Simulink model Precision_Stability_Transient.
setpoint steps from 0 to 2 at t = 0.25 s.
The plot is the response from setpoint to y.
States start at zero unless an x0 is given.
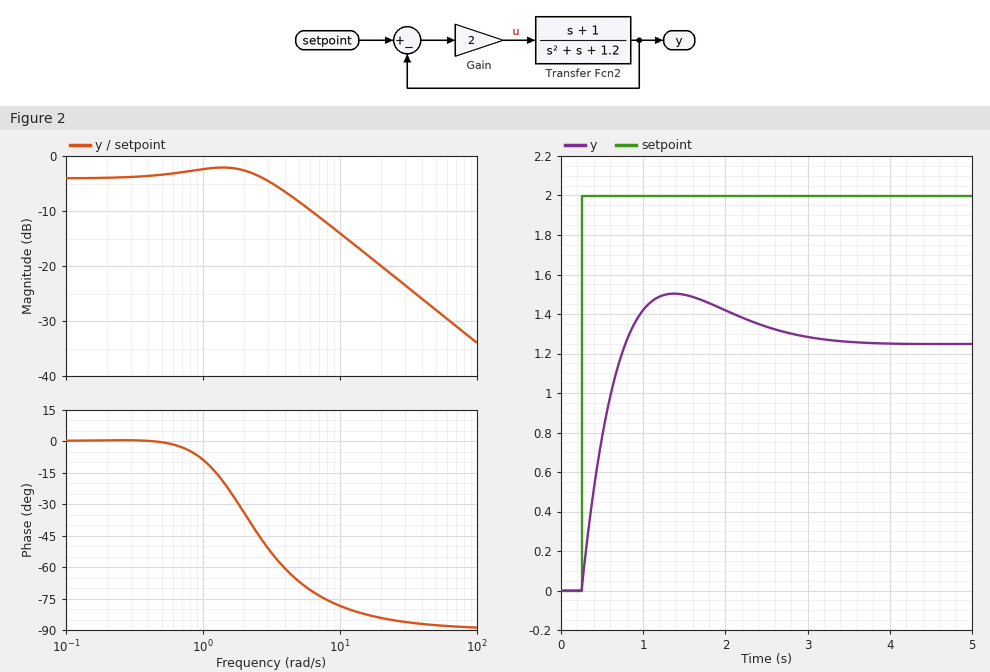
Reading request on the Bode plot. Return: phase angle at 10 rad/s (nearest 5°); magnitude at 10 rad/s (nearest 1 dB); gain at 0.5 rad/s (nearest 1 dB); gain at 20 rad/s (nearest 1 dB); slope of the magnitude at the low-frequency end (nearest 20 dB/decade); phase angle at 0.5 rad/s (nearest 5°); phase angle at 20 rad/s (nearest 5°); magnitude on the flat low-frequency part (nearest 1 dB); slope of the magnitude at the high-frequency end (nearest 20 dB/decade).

-80°
-14 dB
-3 dB
-20 dB
0 dB/decade
0°
-85°
-4 dB
-20 dB/decade
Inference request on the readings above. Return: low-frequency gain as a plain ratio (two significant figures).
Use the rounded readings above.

0.63
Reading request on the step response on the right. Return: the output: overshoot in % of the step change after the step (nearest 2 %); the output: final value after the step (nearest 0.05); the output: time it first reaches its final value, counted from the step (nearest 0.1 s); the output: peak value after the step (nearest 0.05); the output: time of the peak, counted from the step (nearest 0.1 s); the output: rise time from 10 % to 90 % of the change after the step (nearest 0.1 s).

20 %
1.25
0.5 s
1.50
1.1 s
0.4 s
